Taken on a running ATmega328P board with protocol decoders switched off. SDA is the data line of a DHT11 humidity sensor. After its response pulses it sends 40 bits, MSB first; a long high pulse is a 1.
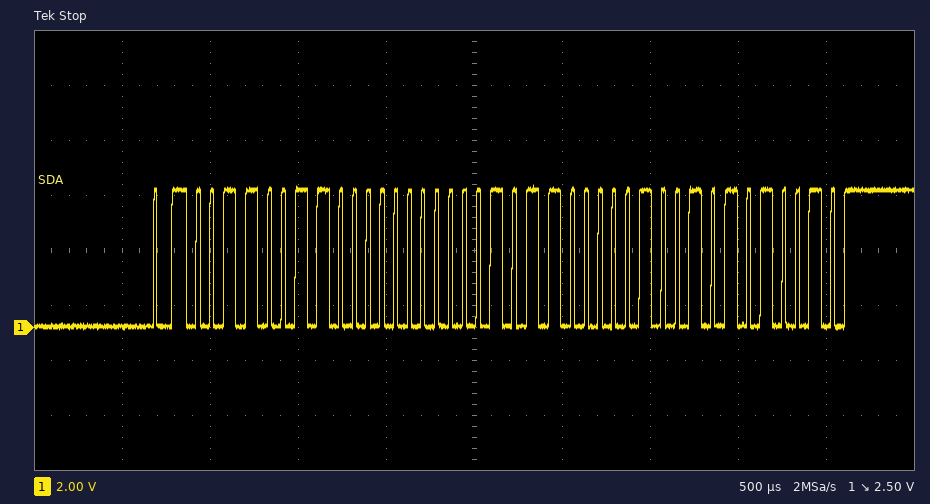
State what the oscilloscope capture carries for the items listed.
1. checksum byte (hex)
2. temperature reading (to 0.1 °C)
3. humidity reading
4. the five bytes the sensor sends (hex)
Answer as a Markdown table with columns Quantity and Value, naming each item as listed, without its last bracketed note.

| Quantity | Value |
|---|---|
| checksum byte | 0x52 |
| temperature reading | 22.9 °C |
| humidity reading | 51 % |
| the five bytes the sensor sends | 33 00 16 09 52 |
